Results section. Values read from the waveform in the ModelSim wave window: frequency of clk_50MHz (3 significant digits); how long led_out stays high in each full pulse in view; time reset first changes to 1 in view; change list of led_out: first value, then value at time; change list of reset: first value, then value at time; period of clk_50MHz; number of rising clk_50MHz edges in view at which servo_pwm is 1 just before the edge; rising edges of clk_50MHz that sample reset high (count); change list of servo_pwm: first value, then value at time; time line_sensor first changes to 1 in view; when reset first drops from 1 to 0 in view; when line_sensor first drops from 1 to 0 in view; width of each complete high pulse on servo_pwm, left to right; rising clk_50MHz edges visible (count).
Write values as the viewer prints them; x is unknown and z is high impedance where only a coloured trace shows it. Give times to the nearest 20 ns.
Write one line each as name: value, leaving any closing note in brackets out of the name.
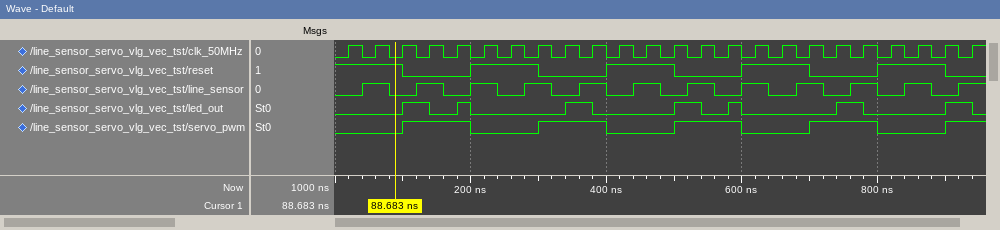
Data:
frequency of clk_50MHz: 25.0 MHz
how long led_out stays high in each full pulse in view: 40 ns, 20 ns, 40 ns, 40 ns, 20 ns, 40 ns, 40 ns
time reset first changes to 1 in view: 200 ns
change list of led_out: first value, then value at time: 0, 1 at 100 ns, 0 at 140 ns, 1 at 180 ns, 0 at 200 ns, 1 at 340 ns, 0 at 380 ns, 1 at 500 ns, 0 at 540 ns, 1 at 580 ns, 0 at 600 ns, 1 at 740 ns, 0 at 780 ns, 1 at 900 ns, 0 at 940 ns
change list of reset: first value, then value at time: 1, 0 at 100 ns, 1 at 200 ns, 0 at 300 ns, 1 at 400 ns, 0 at 500 ns, 1 at 600 ns, 0 at 700 ns, 1 at 800 ns, 0 at 900 ns
period of clk_50MHz: 40 ns
number of rising clk_50MHz edges in view at which servo_pwm is 1 just before the edge: 9
rising edges of clk_50MHz that sample reset high: 15
change list of servo_pwm: first value, then value at time: 0, 1 at 100 ns, 0 at 200 ns, 1 at 300 ns, 0 at 400 ns, 1 at 500 ns, 0 at 600 ns, 1 at 700 ns, 0 at 800 ns, 1 at 900 ns
time line_sensor first changes to 1 in view: 40 ns
when reset first drops from 1 to 0 in view: 100 ns
when line_sensor first drops from 1 to 0 in view: 80 ns
width of each complete high pulse on servo_pwm, left to right: 100 ns, 100 ns, 100 ns, 100 ns
rising clk_50MHz edges visible: 24
